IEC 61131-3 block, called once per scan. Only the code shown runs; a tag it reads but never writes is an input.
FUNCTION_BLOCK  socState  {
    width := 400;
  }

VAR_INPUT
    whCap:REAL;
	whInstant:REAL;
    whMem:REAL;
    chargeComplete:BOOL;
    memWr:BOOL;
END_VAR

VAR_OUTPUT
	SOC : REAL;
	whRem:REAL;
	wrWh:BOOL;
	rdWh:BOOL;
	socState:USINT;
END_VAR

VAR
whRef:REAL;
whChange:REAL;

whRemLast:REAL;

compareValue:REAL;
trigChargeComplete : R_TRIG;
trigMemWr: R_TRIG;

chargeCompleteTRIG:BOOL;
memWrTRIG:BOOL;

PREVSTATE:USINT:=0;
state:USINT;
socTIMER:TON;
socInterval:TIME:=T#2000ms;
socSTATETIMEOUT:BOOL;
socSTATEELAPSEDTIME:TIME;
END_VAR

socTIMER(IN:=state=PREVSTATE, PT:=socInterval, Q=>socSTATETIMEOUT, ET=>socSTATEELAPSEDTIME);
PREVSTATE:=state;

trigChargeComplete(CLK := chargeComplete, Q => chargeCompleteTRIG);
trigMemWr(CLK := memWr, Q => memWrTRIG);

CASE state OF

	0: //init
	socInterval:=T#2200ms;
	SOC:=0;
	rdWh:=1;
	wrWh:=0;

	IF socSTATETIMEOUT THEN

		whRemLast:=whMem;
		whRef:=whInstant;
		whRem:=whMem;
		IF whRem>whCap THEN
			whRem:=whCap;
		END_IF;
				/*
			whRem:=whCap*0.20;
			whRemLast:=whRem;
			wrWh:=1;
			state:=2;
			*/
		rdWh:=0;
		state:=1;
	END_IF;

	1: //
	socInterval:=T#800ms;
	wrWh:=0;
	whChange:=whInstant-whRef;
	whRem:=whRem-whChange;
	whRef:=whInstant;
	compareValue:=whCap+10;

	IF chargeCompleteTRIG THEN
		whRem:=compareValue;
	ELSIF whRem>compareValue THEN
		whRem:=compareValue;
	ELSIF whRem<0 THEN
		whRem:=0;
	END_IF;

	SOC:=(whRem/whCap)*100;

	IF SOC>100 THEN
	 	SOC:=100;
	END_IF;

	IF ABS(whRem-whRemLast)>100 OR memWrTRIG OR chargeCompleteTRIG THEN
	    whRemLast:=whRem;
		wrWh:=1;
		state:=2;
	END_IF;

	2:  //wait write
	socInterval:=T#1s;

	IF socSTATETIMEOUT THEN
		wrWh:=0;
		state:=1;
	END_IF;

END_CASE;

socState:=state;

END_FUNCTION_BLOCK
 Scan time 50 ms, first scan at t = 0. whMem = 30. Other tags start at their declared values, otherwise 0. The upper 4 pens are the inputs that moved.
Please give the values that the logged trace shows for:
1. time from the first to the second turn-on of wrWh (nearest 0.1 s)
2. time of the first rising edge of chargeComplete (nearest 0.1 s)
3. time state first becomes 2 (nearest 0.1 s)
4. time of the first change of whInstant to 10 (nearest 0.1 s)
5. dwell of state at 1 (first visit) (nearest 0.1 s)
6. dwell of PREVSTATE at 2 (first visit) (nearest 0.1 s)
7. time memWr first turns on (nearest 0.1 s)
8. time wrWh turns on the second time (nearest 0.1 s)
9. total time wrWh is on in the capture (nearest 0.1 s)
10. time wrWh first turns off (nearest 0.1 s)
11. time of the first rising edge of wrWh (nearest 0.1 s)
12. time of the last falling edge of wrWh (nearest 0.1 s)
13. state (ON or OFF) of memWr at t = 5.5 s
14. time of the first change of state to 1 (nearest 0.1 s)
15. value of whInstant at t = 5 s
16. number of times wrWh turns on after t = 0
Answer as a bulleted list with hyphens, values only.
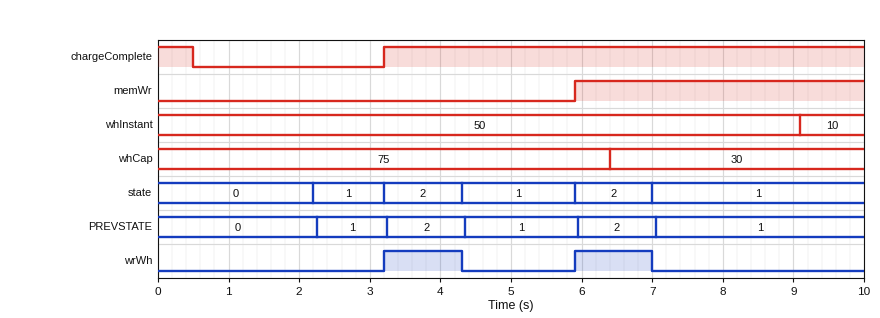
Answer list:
- 2.7 s
- 3.2 s
- 3.2 s
- 9.1 s
- 1.0 s
- 1.1 s
- 5.9 s
- 5.9 s
- 2.2 s
- 4.3 s
- 3.2 s
- 7.0 s
- OFF
- 2.2 s
- 50
- 2
